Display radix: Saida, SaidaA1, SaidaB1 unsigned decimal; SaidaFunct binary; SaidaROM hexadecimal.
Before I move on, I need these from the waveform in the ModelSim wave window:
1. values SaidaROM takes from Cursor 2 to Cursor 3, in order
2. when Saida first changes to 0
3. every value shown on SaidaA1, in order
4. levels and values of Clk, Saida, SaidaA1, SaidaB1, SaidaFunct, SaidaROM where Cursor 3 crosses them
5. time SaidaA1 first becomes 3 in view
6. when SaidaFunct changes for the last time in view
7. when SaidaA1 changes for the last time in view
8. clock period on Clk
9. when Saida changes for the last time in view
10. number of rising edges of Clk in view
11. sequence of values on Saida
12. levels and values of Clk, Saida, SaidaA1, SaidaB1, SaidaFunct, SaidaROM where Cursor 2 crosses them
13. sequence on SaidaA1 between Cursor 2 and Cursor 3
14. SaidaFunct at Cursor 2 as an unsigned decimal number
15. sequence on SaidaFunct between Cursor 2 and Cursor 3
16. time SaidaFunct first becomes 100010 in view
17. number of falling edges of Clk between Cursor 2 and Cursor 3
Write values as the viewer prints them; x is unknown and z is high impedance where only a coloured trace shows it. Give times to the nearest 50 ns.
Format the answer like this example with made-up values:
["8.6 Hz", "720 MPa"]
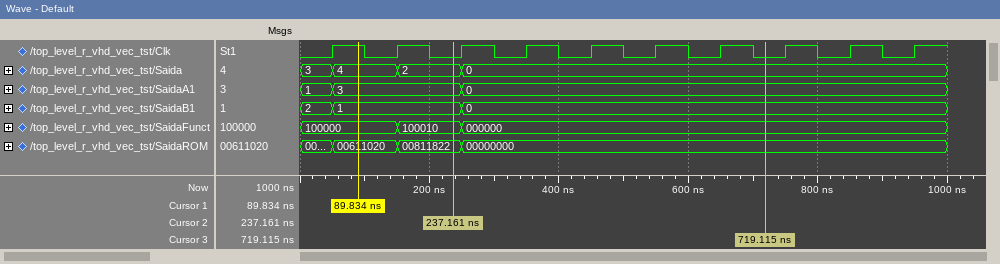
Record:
["00811822, 00000000", "250 ns", "1, 3, 0", "Clk=0, Saida=0, SaidaA1=0, SaidaB1=0, SaidaFunct=000000, SaidaROM=00000000", "50 ns", "250 ns", "250 ns", "100 ns", "250 ns", "10", "3, 4, 2, 0", "Clk=0, Saida=2, SaidaA1=3, SaidaB1=1, SaidaFunct=100010, SaidaROM=00811822", "3, 0", "34", "100010, 000000", "150 ns", "5"]
